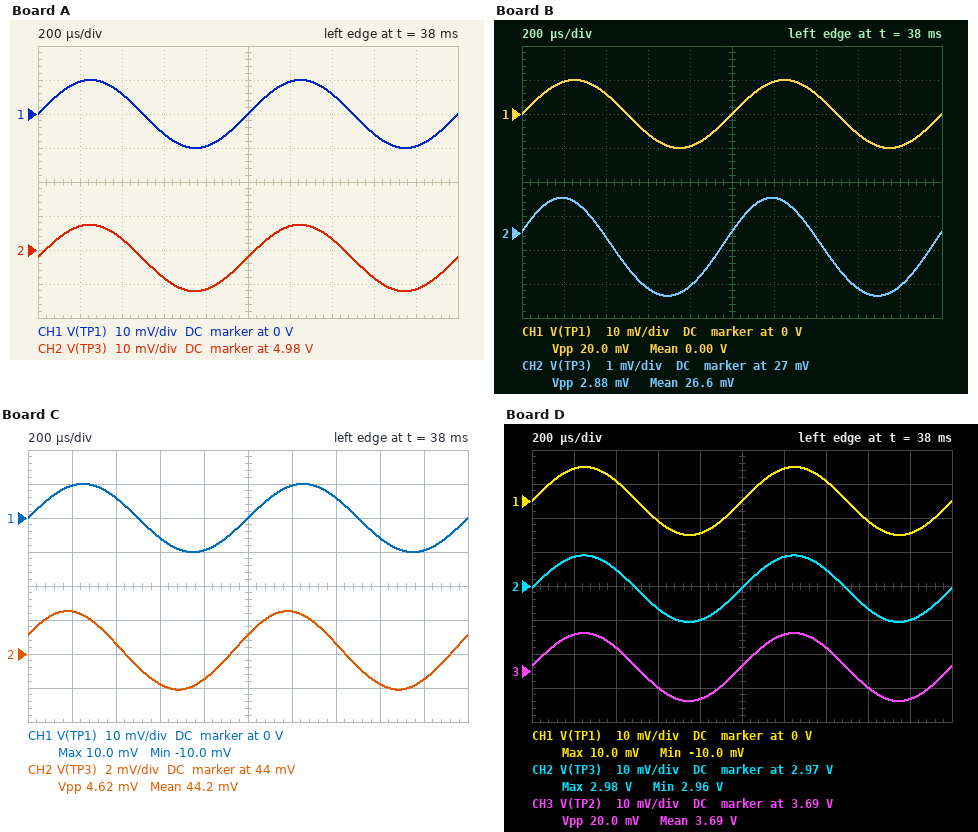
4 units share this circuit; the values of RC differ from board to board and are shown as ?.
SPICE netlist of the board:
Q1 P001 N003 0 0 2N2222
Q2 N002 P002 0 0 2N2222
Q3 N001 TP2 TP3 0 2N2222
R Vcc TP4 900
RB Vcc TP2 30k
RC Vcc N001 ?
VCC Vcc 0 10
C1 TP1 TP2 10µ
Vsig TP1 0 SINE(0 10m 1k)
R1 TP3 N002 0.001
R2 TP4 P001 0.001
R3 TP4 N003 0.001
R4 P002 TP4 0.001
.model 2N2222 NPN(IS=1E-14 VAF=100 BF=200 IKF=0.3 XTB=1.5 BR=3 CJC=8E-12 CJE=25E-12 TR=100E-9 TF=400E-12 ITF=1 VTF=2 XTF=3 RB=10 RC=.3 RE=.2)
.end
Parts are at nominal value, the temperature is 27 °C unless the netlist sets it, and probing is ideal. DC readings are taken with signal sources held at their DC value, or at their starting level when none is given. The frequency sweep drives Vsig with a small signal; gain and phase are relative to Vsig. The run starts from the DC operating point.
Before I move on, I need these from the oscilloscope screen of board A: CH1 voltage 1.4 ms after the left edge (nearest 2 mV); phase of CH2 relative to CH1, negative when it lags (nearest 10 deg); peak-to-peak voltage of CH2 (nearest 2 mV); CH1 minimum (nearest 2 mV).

6 mV
0 deg
20 mV
-10 mV
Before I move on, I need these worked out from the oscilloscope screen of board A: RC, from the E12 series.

470 Ω
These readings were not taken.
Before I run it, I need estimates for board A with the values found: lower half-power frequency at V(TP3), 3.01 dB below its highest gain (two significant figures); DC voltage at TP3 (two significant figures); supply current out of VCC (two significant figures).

22 Hz
5.0 V
21 mA
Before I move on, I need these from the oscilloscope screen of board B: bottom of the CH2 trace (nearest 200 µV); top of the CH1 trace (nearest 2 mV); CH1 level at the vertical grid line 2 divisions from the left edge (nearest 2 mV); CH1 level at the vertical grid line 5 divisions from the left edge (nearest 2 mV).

25.2 mV
10 mV
6 mV
0 V
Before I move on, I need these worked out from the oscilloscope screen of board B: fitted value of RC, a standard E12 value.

3.3 kΩ
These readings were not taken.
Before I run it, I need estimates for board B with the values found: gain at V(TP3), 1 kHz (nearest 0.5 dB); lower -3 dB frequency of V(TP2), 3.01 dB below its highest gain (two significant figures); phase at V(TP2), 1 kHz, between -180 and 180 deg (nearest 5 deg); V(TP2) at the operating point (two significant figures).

-17.0 dB
390 Hz
20 deg
720 mV
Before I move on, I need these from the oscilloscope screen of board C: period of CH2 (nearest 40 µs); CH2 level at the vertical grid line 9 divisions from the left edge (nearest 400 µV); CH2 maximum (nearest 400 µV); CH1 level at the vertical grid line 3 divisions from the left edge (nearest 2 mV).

1.00 ms
42.4 mV
46.4 mV
-6 mV
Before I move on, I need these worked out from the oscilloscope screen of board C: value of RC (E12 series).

1.8 kΩ
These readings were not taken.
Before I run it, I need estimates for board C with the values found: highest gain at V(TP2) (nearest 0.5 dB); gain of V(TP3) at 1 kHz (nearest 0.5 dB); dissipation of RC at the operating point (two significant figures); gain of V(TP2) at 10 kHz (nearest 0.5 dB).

0 dB
-13.0 dB
54 mW
0 dB
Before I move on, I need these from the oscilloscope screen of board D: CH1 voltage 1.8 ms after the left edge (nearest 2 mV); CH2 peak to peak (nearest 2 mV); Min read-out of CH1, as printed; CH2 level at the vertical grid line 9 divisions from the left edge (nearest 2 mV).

-10 mV
20 mV
-10.0 mV
2.960 V
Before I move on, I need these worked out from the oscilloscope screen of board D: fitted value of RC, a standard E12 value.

680 Ω
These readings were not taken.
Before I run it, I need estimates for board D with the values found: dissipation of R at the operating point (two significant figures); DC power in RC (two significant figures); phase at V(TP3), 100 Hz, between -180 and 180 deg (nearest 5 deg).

96 mW
71 mW
10 deg
